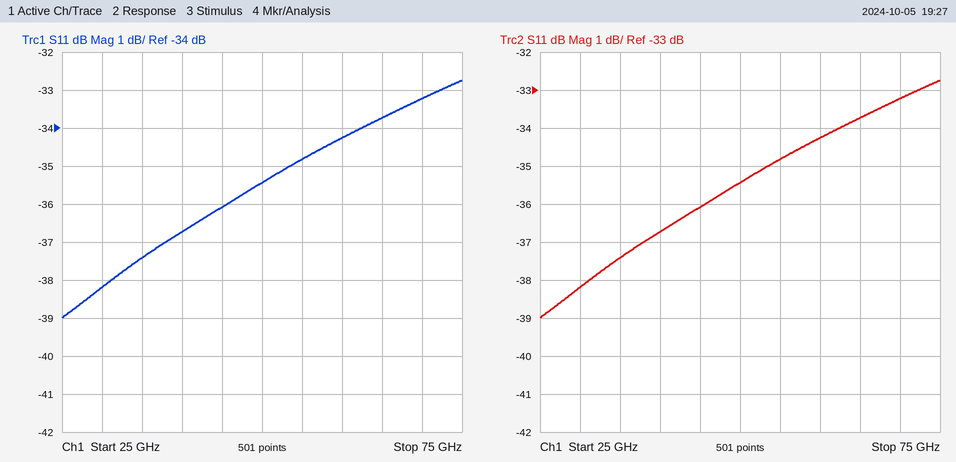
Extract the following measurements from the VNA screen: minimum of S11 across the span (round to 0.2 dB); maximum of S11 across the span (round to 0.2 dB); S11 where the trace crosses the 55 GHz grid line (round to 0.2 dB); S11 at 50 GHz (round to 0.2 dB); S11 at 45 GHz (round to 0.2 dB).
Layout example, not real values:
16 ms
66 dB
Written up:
-39.0 dB
-32.8 dB
-34.8 dB
-35.4 dB
-36.0 dB
